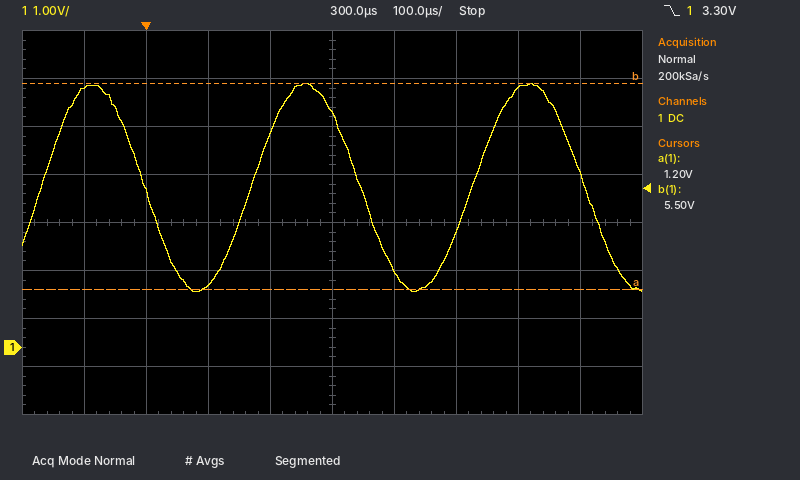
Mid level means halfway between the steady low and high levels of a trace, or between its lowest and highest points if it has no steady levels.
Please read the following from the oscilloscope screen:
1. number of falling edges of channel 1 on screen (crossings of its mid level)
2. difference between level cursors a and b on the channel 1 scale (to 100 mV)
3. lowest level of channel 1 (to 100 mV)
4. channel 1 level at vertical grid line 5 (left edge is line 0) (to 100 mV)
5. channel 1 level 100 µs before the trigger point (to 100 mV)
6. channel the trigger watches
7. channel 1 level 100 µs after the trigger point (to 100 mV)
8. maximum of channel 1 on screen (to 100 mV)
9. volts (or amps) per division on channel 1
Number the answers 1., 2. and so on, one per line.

1. 3
2. 4.3 V
3. 1.2 V
4. 4.9 V
5. 5.4 V
6. channel 1
7. 1.3 V
8. 5.5 V
9. 1 V
